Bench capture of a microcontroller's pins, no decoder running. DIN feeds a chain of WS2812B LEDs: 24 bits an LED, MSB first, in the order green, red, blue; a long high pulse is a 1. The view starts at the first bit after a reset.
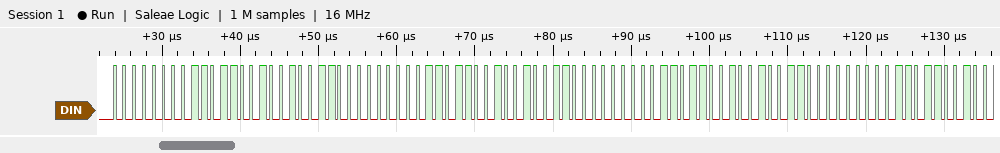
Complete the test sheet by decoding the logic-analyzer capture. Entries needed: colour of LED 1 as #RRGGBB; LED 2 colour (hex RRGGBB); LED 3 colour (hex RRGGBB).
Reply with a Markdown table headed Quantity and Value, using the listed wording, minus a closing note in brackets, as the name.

| Quantity | Value |
|---|---|
| colour of LED 1 as #RRGGBB | #D90026 |
| LED 2 colour | #D90026 |
| LED 3 colour | #D90026 |
